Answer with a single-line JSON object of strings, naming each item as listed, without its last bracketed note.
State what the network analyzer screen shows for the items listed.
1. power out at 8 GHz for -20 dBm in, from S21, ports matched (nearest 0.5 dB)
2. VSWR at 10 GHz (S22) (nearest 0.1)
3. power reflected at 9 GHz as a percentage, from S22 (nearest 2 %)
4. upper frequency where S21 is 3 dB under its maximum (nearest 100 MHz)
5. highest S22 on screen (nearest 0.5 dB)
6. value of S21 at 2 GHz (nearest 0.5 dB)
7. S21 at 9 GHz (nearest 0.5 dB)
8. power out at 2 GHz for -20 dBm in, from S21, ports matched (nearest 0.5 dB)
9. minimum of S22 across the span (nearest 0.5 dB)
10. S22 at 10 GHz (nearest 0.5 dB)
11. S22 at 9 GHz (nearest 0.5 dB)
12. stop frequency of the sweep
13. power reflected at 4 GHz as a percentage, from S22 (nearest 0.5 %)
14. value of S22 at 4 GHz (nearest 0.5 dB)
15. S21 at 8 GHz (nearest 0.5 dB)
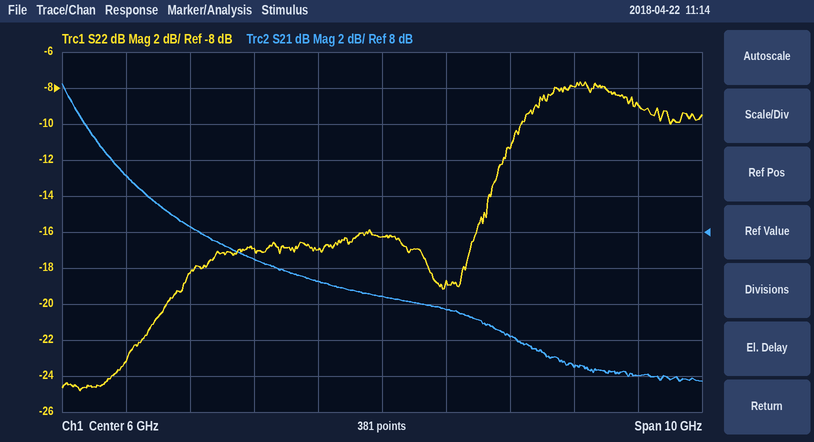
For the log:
{"power out at 8 GHz for -20 dBm in, from S21, ports matched": "-18.0 dBm", "VSWR at 10 GHz (S22)": "2.1", "power reflected at 9 GHz as a percentage, from S22": "16 %", "upper frequency where S21 is 3 dB under its maximum": "1.5 GHz", "highest S22 on screen": "-7.5 dB", "value of S21 at 2 GHz": "11.0 dB", "S21 at 9 GHz": "0.5 dB", "power out at 2 GHz for -20 dBm in, from S21, ports matched": "-9.0 dBm", "minimum of S22 across the span": "-25.0 dB", "S22 at 10 GHz": "-9.0 dB", "S22 at 9 GHz": "-8.0 dB", "stop frequency of the sweep": "11 GHz", "power reflected at 4 GHz as a percentage, from S22": "2.0 %", "value of S22 at 4 GHz": "-17.0 dB", "S21 at 8 GHz": "2.0 dB"}
